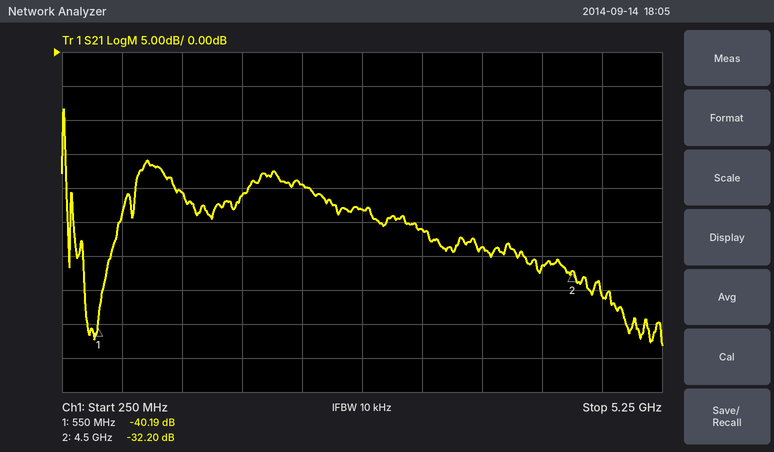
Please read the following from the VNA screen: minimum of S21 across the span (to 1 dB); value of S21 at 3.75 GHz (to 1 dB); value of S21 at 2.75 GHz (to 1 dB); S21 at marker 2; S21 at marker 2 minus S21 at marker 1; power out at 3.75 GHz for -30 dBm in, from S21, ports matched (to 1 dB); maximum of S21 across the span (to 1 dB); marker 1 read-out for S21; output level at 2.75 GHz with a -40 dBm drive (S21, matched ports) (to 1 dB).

-43 dB
-29 dB
-23 dB
-32.20 dB
7.99 dB
-59 dBm
-8 dB
-40.19 dB
-63 dBm
